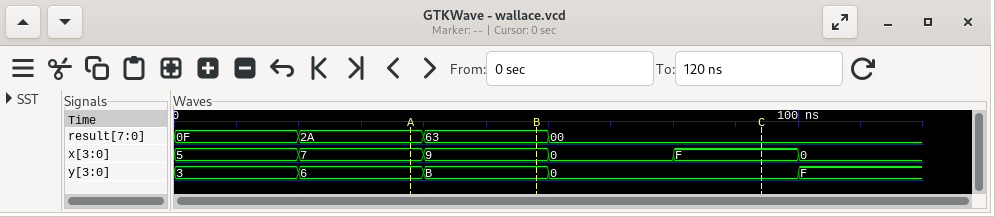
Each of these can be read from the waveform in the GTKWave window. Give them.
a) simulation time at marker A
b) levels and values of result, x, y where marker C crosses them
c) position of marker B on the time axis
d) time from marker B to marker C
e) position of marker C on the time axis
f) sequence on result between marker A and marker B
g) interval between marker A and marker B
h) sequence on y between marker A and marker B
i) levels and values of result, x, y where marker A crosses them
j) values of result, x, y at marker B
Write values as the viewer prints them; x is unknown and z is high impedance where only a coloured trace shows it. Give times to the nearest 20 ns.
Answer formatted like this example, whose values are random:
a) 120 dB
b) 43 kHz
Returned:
a) 40 ns
b) result=00, x=F, y=0
c) 60 ns
d) 40 ns
e) 100 ns
f) 2A, 63
g) 20 ns
h) 6, B
i) result=2A, x=7, y=6
j) result=63, x=9, y=B
